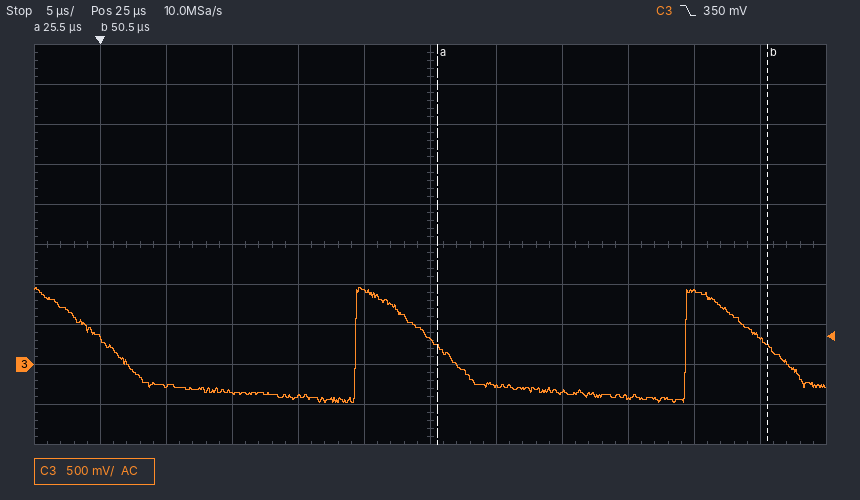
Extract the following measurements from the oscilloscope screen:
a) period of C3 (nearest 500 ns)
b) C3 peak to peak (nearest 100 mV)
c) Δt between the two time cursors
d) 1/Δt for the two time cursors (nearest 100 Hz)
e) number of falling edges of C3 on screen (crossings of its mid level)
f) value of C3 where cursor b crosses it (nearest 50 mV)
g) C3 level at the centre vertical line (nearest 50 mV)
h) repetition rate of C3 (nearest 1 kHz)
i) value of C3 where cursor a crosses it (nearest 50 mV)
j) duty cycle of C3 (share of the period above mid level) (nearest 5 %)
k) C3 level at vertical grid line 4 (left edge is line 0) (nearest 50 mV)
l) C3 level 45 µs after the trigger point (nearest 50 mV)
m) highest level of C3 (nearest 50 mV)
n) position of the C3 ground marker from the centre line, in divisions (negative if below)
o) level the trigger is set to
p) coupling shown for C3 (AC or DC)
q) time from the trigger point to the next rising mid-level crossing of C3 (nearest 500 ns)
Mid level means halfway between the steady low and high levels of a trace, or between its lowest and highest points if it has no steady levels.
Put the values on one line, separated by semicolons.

25.0 µs; 1.40 V; 25.0 µs; 40.0 kHz; 3; 250 mV; 300 mV; 40 kHz; 200 mV; 25 %; -400 mV; 900 mV; 950 mV; -3.0 div; 350 mV; AC; 19.5 µs
